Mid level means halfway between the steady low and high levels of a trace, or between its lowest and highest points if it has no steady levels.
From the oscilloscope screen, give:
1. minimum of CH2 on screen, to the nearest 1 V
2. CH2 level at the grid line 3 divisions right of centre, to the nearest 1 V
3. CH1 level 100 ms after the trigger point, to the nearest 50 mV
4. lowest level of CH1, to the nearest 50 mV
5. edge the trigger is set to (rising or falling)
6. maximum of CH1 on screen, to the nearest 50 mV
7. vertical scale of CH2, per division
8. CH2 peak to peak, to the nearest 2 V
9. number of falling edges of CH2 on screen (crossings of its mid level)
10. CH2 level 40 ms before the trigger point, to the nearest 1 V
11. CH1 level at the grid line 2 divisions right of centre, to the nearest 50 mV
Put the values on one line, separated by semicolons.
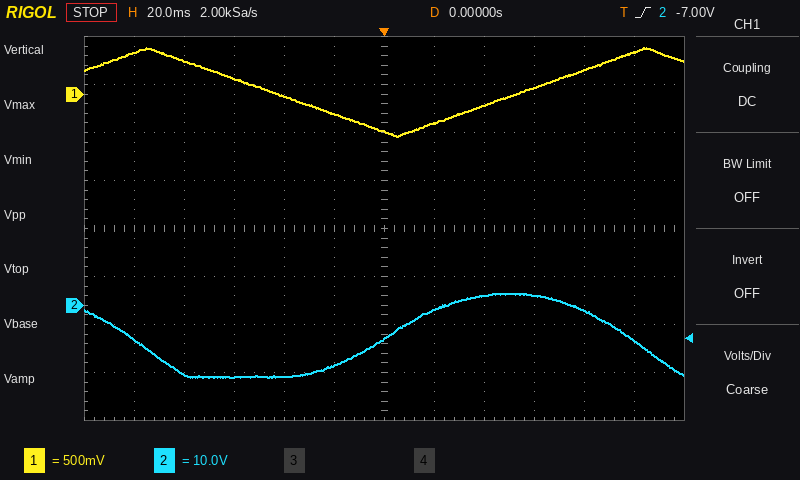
-15 V; 2 V; 450 mV; -450 mV; rising; 500 mV; 10 V; 18 V; 2; -15 V; -100 mV
